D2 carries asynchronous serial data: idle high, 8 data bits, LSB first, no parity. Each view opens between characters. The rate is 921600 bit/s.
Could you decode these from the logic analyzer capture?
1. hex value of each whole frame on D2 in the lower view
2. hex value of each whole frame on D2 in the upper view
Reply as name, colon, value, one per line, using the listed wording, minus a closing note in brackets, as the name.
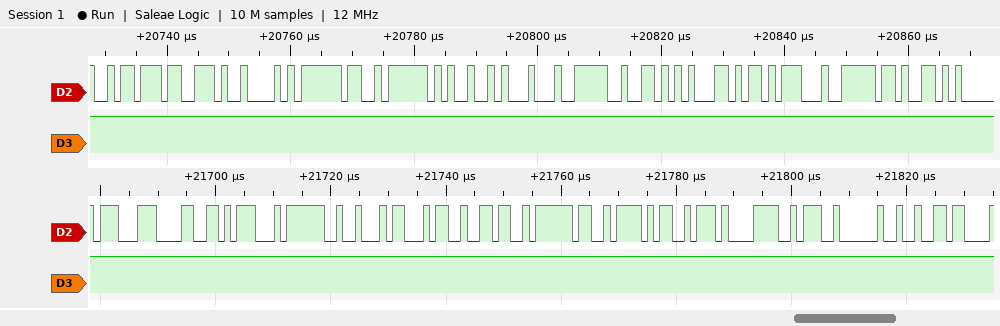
hex value of each whole frame on D2 in the lower view: C7, 98, 1D, 3F, A2, 34, 36, BF, 7A, D3, E1, 3A, 20, B2
hex value of each whole frame on D2 in the upper view: DA, 73, 42, BF, FA, 25, 11, 3E, 56, AC, 1D, BE, 59
